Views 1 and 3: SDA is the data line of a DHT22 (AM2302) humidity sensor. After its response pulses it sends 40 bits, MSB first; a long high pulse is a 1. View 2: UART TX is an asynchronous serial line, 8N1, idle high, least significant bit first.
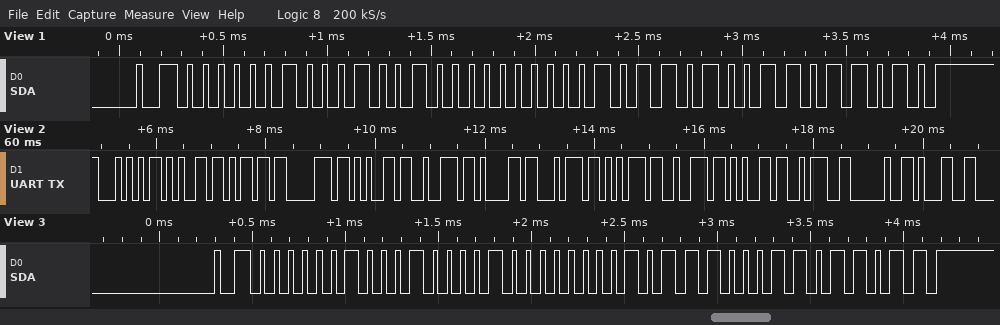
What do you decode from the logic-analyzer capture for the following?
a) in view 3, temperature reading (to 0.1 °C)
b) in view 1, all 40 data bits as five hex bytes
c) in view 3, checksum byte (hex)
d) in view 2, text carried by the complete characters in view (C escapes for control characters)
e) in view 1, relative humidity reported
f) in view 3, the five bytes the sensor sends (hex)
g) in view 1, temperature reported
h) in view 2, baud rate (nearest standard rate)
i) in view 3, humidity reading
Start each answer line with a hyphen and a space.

- 18.4 °C
- 02 24 00 B4 DA
- 0xDB
- "Temperature: 1"
- 54.8 %
- 02 21 00 B8 DB
- 18.0 °C
- 9600 baud
- 54.5 %
